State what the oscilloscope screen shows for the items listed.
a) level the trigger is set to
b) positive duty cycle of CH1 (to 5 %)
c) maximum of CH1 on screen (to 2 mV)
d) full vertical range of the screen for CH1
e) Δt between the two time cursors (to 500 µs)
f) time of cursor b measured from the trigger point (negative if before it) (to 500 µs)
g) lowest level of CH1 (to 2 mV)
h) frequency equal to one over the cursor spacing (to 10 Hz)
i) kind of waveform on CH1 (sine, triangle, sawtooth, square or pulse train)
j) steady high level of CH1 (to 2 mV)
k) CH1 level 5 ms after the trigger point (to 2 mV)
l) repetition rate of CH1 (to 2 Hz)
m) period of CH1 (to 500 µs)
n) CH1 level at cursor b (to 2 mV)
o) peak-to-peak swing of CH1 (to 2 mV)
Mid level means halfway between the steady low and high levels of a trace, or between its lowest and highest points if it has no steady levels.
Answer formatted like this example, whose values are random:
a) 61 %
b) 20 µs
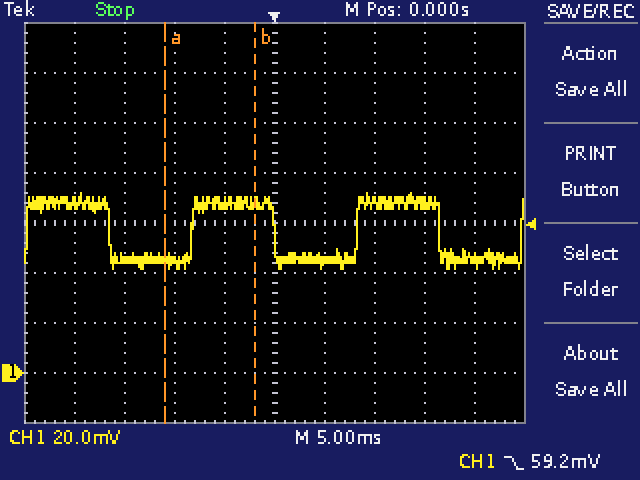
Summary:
a) 59.2 mV
b) 50 %
c) 72 mV
d) 160 mV
e) 9.0 ms
f) -2.0 ms
g) 42 mV
h) 110 Hz
i) square
j) 68 mV
k) 44 mV
l) 60 Hz
m) 16.5 ms
n) 68 mV
o) 30 mV
